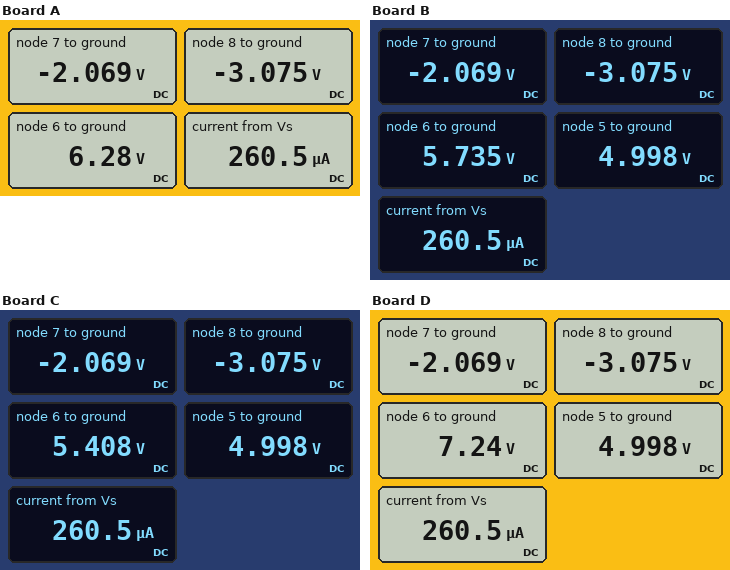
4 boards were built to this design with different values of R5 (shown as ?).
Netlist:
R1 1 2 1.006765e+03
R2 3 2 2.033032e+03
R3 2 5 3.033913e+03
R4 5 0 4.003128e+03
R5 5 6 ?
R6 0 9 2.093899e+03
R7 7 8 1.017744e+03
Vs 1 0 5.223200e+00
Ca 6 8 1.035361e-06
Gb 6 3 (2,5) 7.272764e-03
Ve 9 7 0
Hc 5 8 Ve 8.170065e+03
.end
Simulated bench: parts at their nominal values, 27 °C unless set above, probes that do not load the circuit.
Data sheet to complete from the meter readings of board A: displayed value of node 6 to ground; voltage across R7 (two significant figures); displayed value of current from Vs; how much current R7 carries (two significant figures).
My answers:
6.28 V
1.0 V
260.5 µA
990 µA
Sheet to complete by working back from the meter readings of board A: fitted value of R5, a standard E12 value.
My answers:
4.7 kΩ
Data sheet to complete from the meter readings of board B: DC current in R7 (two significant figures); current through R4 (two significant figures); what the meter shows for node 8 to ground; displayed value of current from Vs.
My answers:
990 µA
1.2 mA
-3.075 V
260.5 µA
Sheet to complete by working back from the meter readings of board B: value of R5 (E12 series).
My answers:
2.7 kΩ
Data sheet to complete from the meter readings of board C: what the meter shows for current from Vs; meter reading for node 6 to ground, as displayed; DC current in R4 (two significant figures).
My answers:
260.5 µA
5.408 V
1.2 mA
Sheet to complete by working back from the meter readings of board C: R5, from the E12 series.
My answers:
1.5 kΩ
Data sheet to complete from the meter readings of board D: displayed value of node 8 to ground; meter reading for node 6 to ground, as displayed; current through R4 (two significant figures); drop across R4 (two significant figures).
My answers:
-3.075 V
7.24 V
1.2 mA
5.0 V
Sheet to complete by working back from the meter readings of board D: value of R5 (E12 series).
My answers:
8.2 kΩ
